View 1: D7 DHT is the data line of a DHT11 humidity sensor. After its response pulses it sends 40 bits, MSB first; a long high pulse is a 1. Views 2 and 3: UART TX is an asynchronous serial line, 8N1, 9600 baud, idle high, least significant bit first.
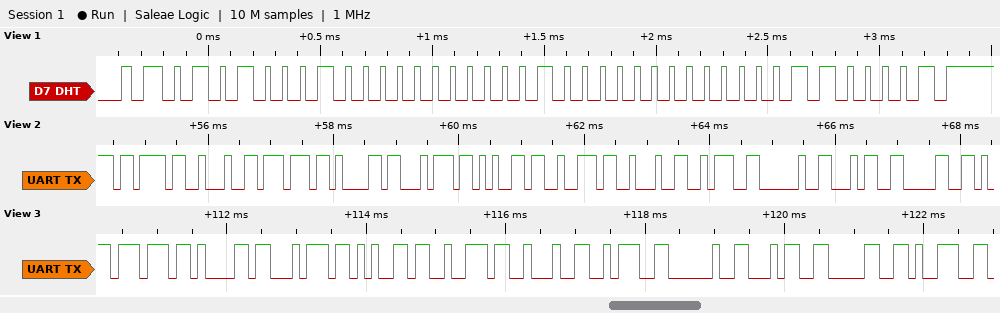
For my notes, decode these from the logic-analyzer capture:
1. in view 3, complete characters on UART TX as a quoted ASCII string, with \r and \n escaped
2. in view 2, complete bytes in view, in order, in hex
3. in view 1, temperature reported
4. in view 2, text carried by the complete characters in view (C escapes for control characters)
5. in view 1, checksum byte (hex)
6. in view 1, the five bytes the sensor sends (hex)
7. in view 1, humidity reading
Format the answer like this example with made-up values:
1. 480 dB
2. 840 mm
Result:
1. "water\": 409"
2. 7B 22 77 61 74 65 72 22 3A 20 34 30
3. 16.0 °C
4. "{\"water\": 40"
5. 0x61
6. 51 00 10 00 61
7. 81 %
